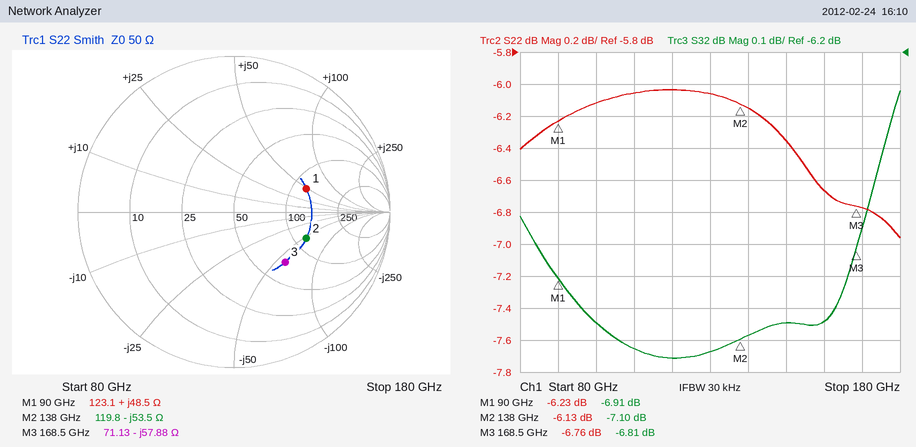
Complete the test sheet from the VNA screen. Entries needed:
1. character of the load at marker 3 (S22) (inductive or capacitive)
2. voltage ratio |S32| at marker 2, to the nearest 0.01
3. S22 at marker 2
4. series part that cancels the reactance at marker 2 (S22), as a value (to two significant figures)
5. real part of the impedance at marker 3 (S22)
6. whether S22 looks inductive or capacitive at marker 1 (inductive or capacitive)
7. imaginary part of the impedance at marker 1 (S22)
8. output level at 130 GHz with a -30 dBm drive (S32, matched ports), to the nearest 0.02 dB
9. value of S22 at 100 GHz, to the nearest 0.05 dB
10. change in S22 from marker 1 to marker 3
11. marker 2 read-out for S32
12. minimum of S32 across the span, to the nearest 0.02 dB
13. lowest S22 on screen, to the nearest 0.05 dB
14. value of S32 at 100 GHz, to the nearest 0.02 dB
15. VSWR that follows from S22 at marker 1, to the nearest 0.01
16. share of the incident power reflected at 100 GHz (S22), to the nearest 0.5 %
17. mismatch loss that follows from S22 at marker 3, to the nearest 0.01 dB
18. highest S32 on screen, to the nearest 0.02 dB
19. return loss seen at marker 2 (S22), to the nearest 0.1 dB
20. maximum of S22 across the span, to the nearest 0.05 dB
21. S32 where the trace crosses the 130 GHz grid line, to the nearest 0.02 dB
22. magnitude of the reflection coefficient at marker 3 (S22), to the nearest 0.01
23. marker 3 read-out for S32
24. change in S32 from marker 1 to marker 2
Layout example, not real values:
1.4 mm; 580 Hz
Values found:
capacitive; 0.44; -6.13 dB; 62 pH; 71.13 Ω; inductive; +48.5 Ω; -37.14 dBm; -6.10 dB; -0.53 dB; -7.10 dB; -7.16 dB; -6.95 dB; -7.04 dB; 2.91; 24.5 %; 1.03 dB; -6.32 dB; 6.1 dB; -6.05 dB; -7.14 dB; 0.46; -6.81 dB; -0.19 dB
